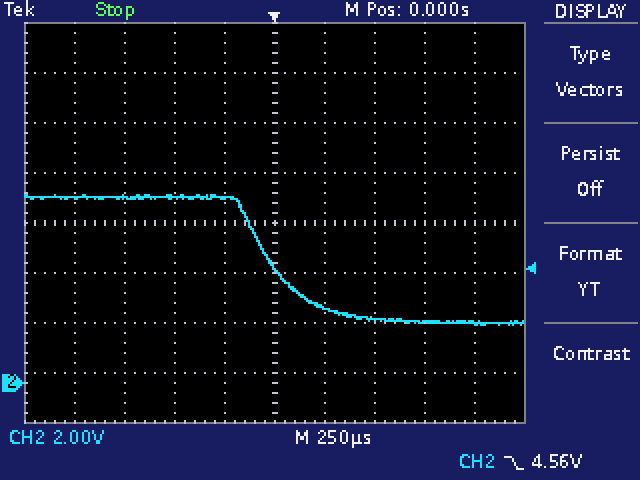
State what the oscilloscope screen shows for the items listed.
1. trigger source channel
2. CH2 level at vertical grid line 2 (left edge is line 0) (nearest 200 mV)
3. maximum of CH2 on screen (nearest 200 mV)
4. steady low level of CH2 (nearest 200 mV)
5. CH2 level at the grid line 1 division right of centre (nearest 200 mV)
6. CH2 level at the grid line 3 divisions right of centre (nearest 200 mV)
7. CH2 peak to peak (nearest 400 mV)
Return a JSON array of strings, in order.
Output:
["CH2", "7.4 V", "7.6 V", "2.4 V", "3.0 V", "2.4 V", "5.2 V"]
